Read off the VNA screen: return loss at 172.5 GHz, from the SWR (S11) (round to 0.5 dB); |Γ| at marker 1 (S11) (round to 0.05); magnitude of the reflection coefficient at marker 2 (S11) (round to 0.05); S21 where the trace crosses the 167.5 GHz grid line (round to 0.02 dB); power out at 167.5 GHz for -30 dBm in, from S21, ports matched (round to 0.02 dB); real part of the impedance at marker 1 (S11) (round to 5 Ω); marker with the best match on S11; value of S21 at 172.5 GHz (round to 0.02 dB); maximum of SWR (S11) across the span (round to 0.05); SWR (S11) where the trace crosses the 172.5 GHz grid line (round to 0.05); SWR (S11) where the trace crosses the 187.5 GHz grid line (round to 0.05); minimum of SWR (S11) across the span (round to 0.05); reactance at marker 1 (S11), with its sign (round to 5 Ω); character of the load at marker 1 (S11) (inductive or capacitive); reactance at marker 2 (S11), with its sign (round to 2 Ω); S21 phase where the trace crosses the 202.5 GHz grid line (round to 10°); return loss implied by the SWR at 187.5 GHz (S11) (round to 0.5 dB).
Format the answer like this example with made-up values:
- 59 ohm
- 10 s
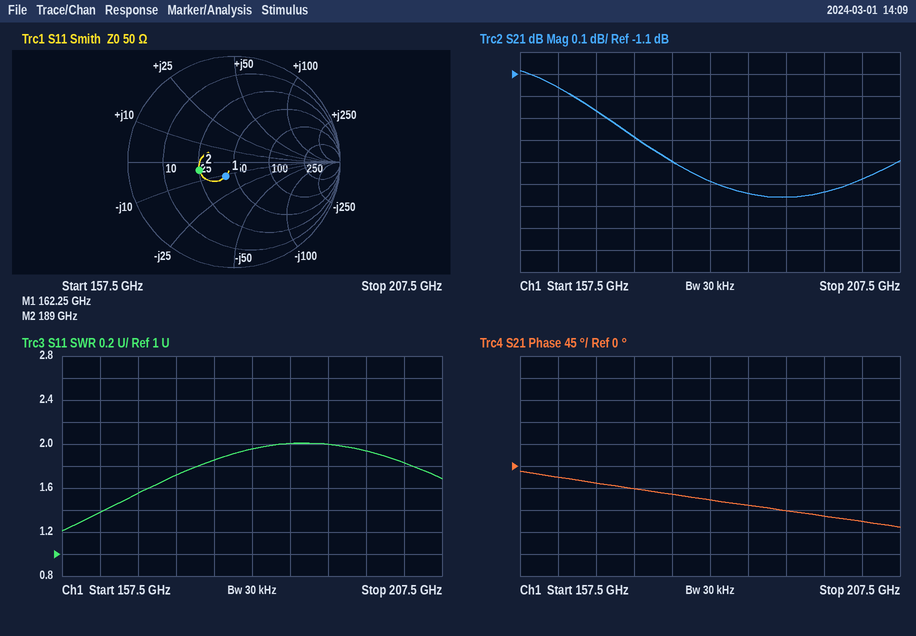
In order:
- 11.5 dB
- 0.15
- 0.35
- -1.26 dB
- -31.26 dBm
- 40 Ω
- marker 1
- -1.38 dB
- 2.00
- 1.70
- 2.00
- 1.20
- -10 Ω
- capacitive
- -4 Ω
- -110°
- 9.5 dB
